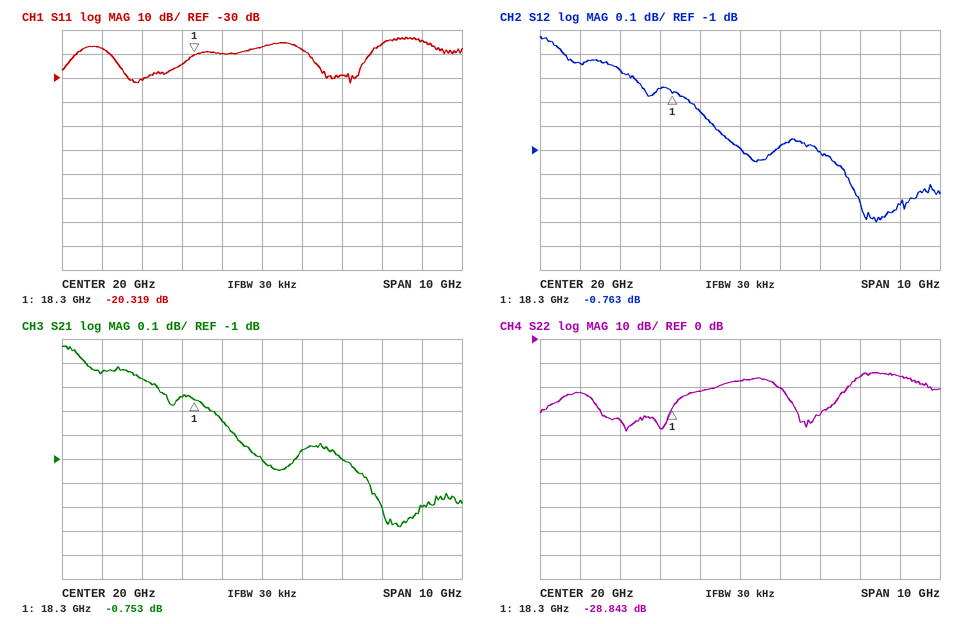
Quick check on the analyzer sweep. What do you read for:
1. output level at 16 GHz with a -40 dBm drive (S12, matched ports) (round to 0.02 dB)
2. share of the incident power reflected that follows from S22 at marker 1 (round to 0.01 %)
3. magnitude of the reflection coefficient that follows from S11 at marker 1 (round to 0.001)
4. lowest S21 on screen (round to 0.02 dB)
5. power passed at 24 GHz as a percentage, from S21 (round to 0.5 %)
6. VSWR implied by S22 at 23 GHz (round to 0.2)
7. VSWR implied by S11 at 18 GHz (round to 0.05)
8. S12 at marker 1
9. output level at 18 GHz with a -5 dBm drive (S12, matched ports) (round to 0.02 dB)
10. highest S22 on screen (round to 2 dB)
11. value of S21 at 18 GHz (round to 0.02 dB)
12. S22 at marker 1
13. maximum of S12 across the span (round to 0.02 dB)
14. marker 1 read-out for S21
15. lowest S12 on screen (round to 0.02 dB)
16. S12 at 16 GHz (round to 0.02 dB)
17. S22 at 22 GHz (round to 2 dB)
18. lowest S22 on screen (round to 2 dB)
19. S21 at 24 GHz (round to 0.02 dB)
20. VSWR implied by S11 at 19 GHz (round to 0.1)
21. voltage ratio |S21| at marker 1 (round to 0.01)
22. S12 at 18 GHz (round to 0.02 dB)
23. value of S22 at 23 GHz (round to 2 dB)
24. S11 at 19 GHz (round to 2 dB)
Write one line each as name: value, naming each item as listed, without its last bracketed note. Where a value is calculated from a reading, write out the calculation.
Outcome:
output level at 16 GHz with a -40 dBm drive (S12, matched ports): -40 dBm + (-0.64 dB) = -40.64 dBm
share of the incident power reflected that follows from S22 at marker 1: 10^(-28.843/10) ≈ 0.13 %
magnitude of the reflection coefficient that follows from S11 at marker 1: 10^(-20.319/20) ≈ 0.096
lowest S21 on screen: -1.28 dB
power passed at 24 GHz as a percentage, from S21: 10^(-1.2/10) ≈ 75.9 %, so 76.0 % to the nearest 0.5 %
VSWR implied by S22 at 23 GHz: |Γ| = 10^(-16/20) = 0.1585; VSWR = (1 + 0.1585)/(1 − 0.1585) ≈ 1.4
VSWR implied by S11 at 18 GHz: |Γ| = 10^(-24/20) = 0.0631; VSWR = (1 + 0.0631)/(1 − 0.0631) ≈ 1.13, so 1.15 to the nearest 0.05
S12 at marker 1: -0.763 dB
output level at 18 GHz with a -5 dBm drive (S12, matched ports): -5 dBm + (-0.74 dB) = -5.74 dBm
highest S22 on screen: -14 dB
value of S21 at 18 GHz: -0.74 dB
S22 at marker 1: -28.843 dB
maximum of S12 across the span: -0.52 dB
marker 1 read-out for S21: -0.753 dB
lowest S12 on screen: -1.30 dB
S12 at 16 GHz: -0.64 dB
S22 at 22 GHz: -32 dB
lowest S22 on screen: -38 dB
S21 at 24 GHz: -1.20 dB
VSWR implied by S11 at 19 GHz: |Γ| = 10^(-20/20) = 0.1000; VSWR = (1 + 0.1000)/(1 − 0.1000) ≈ 1.2
voltage ratio |S21| at marker 1: 10^(-0.753/20) ≈ 0.92
S12 at 18 GHz: -0.74 dB
value of S22 at 23 GHz: -16 dB
S11 at 19 GHz: -20 dB
